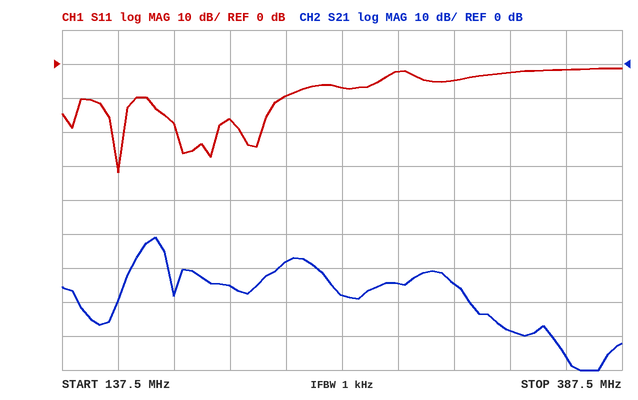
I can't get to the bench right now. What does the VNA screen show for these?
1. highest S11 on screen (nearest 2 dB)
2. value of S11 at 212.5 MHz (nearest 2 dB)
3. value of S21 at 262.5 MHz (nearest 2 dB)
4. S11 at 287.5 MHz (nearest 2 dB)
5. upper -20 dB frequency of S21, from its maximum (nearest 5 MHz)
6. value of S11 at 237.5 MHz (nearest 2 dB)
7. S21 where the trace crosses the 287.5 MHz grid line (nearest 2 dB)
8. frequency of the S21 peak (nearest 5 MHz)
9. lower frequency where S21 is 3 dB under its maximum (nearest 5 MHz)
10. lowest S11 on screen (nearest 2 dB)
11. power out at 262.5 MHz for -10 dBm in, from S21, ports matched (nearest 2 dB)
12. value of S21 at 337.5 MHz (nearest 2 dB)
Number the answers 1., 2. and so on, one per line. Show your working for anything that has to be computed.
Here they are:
1. -2 dB
2. -16 dB
3. -68 dB
4. -2 dB
5. 320 MHz
6. -10 dB
7. -64 dB
8. 180 MHz
9. 175 MHz
10. -32 dB
11. -10 dBm + (-68 dB) = -78 dBm
12. -78 dB
